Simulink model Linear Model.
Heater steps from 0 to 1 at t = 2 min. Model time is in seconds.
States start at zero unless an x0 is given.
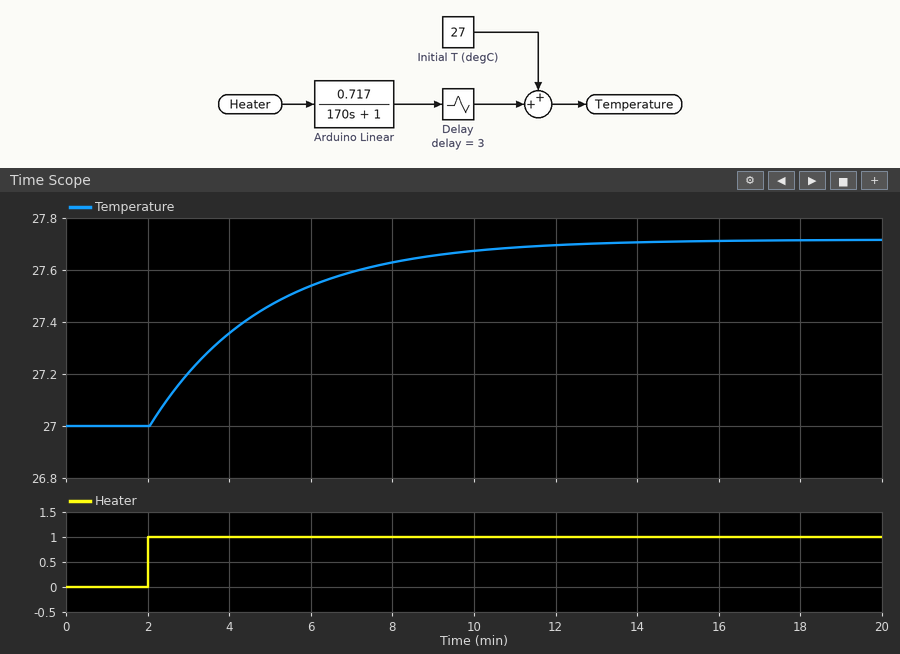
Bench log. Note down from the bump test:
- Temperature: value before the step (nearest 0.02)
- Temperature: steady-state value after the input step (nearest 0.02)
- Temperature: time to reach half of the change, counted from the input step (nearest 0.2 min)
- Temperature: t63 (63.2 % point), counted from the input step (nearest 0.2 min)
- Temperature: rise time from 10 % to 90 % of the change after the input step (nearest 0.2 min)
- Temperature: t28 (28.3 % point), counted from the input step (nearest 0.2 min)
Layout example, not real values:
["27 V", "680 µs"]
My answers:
["27.00", "27.72", "2.0 min", "2.8 min", "6.2 min", "1.0 min"]
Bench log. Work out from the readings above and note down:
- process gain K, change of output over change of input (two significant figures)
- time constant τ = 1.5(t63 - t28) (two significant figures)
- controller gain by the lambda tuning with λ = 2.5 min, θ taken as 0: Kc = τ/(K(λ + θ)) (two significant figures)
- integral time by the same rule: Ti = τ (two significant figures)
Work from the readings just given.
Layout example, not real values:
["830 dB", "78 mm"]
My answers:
["0.72", "2.7 min", "1.5", "2.7 min"]
